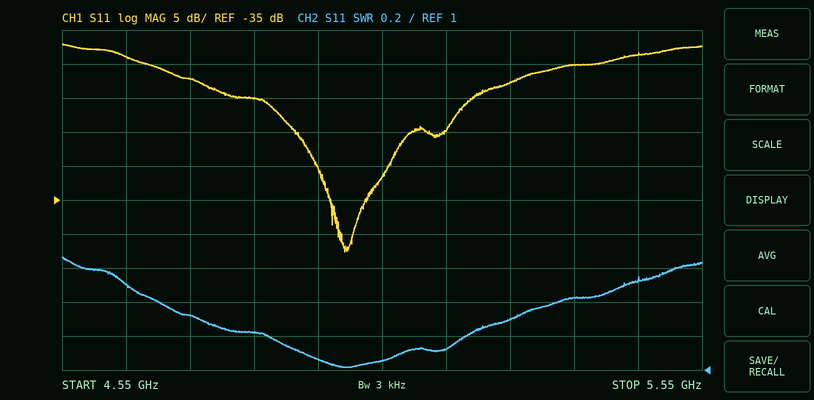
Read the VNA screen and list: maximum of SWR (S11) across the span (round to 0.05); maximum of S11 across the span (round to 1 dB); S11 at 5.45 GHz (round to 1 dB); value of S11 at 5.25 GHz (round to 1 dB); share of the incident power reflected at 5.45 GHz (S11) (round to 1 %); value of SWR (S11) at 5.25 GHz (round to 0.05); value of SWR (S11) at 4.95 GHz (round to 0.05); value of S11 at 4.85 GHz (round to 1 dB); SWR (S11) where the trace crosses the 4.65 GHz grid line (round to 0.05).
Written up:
1.65
-12 dB
-14 dB
-18 dB
4 %
1.30
1.05
-20 dB
1.50
